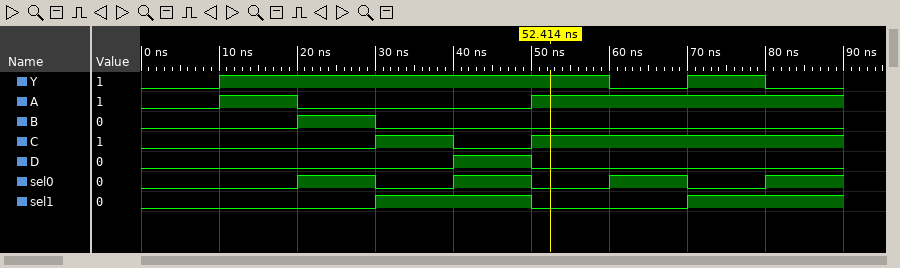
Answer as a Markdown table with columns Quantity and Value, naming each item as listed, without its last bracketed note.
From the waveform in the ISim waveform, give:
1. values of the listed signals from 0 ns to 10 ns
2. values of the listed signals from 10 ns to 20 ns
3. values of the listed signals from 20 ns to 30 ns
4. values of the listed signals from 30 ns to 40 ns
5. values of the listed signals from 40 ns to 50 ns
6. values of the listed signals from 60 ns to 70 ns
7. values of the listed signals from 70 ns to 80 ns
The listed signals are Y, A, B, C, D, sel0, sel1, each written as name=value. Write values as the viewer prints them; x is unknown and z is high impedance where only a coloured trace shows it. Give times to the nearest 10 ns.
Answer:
| Quantity | Value |
|---|---|
| values of the listed signals from 0 ns to 10 ns | Y=0, A=0, B=0, C=0, D=0, sel0=0, sel1=0 |
| values of the listed signals from 10 ns to 20 ns | Y=1, A=1, B=0, C=0, D=0, sel0=0, sel1=0 |
| values of the listed signals from 20 ns to 30 ns | Y=1, A=0, B=1, C=0, D=0, sel0=1, sel1=0 |
| values of the listed signals from 30 ns to 40 ns | Y=1, A=0, B=0, C=1, D=0, sel0=0, sel1=1 |
| values of the listed signals from 40 ns to 50 ns | Y=1, A=0, B=0, C=0, D=1, sel0=1, sel1=1 |
| values of the listed signals from 60 ns to 70 ns | Y=0, A=1, B=0, C=1, D=0, sel0=1, sel1=0 |
| values of the listed signals from 70 ns to 80 ns | Y=1, A=1, B=0, C=1, D=0, sel0=0, sel1=1 |
